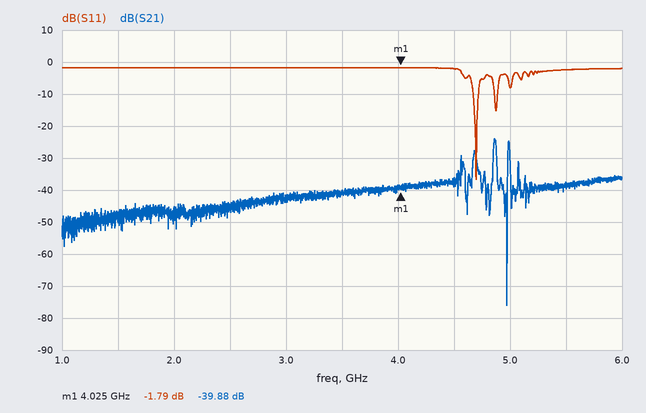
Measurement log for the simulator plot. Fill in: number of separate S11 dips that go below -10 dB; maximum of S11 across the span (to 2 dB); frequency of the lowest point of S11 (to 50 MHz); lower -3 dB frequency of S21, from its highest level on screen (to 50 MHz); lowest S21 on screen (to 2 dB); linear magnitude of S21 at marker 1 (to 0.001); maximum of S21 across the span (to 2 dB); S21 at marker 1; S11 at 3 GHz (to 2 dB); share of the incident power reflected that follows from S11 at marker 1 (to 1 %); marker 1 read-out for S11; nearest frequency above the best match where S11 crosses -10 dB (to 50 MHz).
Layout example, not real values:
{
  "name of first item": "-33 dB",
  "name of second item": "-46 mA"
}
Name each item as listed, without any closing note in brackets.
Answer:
{
  "number of separate S11 dips that go below -10 dB": "2",
  "maximum of S11 across the span": "-2 dB",
  "frequency of the lowest point of S11": "4.70 GHz",
  "lower -3 dB frequency of S21, from its highest level on screen": "4.85 GHz",
  "lowest S21 on screen": "-76 dB",
  "linear magnitude of S21 at marker 1": "0.010",
  "maximum of S21 across the span": "-24 dB",
  "S21 at marker 1": "-39.88 dB",
  "S11 at 3 GHz": "-2 dB",
  "share of the incident power reflected that follows from S11 at marker 1": "66 %",
  "marker 1 read-out for S11": "-1.79 dB",
  "nearest frequency above the best match where S11 crosses -10 dB": "4.70 GHz"
}
